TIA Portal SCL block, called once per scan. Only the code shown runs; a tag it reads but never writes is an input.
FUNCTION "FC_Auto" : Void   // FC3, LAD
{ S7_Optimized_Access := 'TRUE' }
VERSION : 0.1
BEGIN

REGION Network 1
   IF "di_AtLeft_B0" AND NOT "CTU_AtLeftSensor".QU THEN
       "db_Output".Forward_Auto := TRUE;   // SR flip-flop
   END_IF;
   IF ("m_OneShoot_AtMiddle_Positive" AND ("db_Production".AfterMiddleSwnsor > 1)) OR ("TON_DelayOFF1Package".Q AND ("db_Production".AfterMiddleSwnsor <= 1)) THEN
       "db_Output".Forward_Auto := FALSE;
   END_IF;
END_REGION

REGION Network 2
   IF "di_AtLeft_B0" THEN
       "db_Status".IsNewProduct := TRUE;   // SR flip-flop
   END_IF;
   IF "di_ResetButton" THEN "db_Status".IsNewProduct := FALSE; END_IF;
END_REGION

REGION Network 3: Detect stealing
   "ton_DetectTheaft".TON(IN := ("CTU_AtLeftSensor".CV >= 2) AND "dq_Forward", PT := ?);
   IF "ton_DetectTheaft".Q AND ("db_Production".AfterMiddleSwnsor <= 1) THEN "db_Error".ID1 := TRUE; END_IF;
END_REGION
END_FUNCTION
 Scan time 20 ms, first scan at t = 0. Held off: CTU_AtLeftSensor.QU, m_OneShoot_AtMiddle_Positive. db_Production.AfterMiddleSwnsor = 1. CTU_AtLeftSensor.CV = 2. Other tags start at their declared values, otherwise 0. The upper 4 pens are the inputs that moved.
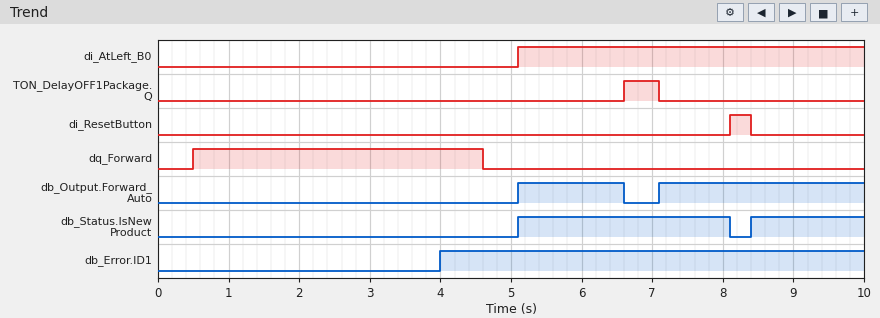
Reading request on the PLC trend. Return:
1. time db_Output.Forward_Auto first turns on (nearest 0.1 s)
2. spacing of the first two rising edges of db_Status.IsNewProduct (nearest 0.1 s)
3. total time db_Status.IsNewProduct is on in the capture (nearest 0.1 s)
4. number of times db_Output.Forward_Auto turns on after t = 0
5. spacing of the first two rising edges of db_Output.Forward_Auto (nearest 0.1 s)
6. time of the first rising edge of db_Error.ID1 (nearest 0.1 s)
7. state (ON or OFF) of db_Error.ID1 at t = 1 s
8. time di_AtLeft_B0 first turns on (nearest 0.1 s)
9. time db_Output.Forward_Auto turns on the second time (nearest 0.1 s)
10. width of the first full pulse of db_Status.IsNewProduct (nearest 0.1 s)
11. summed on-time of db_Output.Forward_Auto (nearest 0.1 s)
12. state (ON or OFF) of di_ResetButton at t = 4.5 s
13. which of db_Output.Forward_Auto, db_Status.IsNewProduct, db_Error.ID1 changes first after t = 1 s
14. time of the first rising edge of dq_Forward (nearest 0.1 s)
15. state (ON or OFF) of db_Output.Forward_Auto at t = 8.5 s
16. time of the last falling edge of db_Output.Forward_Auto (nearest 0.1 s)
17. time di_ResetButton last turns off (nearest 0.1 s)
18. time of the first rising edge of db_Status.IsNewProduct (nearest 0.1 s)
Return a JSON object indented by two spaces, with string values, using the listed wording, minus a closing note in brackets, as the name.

{
  "time db_Output.Forward_Auto first turns on": "5.1 s",
  "spacing of the first two rising edges of db_Status.IsNewProduct": "3.3 s",
  "total time db_Status.IsNewProduct is on in the capture": "4.6 s",
  "number of times db_Output.Forward_Auto turns on after t = 0": "2",
  "spacing of the first two rising edges of db_Output.Forward_Auto": "2.0 s",
  "time of the first rising edge of db_Error.ID1": "4.0 s",
  "state (ON or OFF) of db_Error.ID1 at t = 1 s": "OFF",
  "time di_AtLeft_B0 first turns on": "5.1 s",
  "time db_Output.Forward_Auto turns on the second time": "7.1 s",
  "width of the first full pulse of db_Status.IsNewProduct": "3.0 s",
  "summed on-time of db_Output.Forward_Auto": "4.4 s",
  "state (ON or OFF) of di_ResetButton at t = 4.5 s": "OFF",
  "which of db_Output.Forward_Auto, db_Status.IsNewProduct, db_Error.ID1 changes first after t = 1 s": "db_Error.ID1",
  "time of the first rising edge of dq_Forward": "0.5 s",
  "state (ON or OFF) of db_Output.Forward_Auto at t = 8.5 s": "ON",
  "time of the last falling edge of db_Output.Forward_Auto": "6.6 s",
  "time di_ResetButton last turns off": "8.4 s",
  "time of the first rising edge of db_Status.IsNewProduct": "5.1 s"
}
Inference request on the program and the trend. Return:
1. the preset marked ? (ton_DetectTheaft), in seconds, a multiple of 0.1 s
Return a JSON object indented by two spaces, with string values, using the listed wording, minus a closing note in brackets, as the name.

{
  "the preset marked ? (ton_DetectTheaft), in seconds, a multiple of 0.1 s": "3.5 s"
}
